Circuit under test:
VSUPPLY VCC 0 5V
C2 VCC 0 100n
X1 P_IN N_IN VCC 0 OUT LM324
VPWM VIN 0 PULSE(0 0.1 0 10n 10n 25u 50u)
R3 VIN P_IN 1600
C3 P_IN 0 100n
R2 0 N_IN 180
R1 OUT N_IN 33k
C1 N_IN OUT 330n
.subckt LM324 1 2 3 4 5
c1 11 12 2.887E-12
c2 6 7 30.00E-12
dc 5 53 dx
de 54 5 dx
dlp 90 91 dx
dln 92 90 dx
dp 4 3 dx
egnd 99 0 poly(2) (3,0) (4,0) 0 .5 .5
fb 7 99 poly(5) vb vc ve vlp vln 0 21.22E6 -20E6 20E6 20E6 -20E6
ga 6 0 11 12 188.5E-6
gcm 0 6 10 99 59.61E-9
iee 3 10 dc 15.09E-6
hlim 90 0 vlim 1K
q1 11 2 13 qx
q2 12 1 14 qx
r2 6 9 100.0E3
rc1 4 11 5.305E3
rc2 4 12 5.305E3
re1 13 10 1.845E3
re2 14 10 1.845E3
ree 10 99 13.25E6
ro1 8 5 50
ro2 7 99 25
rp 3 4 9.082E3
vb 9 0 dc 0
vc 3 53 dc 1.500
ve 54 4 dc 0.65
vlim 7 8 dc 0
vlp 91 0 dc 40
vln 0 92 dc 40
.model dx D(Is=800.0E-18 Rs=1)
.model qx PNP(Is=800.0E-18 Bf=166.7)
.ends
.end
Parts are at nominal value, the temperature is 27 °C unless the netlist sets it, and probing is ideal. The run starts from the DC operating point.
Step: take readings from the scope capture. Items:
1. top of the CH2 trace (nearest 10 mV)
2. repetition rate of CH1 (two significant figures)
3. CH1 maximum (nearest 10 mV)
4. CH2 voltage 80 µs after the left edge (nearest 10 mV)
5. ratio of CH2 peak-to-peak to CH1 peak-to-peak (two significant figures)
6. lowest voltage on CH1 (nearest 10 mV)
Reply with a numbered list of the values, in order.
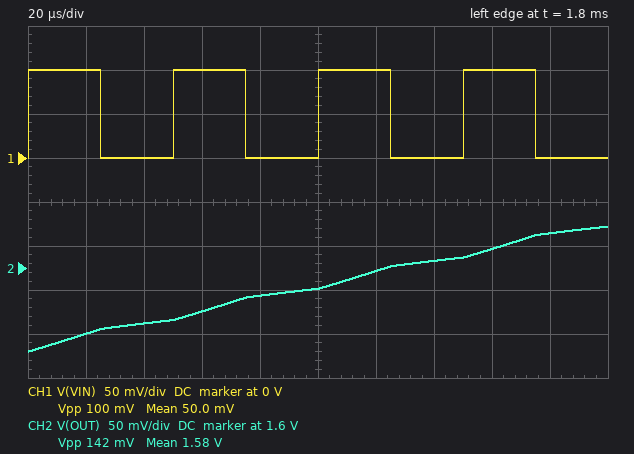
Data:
1. 1.65 V
2. 20 kHz
3. 100 mV
4. 1.57 V
5. 1.4
6. 0 V
